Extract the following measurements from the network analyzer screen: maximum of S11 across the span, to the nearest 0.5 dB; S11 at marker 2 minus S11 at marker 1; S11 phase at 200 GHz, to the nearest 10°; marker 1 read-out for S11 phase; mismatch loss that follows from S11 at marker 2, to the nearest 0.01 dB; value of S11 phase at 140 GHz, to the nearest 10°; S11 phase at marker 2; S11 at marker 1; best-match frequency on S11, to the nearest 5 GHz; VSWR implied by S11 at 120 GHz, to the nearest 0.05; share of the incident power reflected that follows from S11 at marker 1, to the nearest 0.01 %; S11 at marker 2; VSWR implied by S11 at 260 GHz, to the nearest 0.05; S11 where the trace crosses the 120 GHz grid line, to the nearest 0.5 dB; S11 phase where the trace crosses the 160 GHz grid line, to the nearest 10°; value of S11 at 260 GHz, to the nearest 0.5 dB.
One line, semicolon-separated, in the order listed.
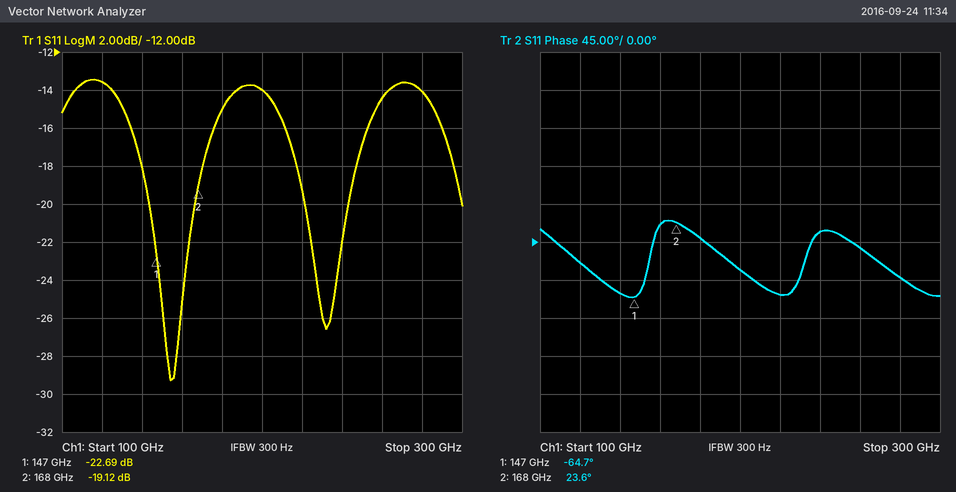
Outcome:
-13.5 dB; 3.57 dB; -30°; -64.7°; 0.05 dB; -60°; 23.6°; -22.69 dB; 155 GHz; 1.55; 0.54 %; -19.12 dB; 1.45; -13.5 dB; 20°; -14.5 dB
